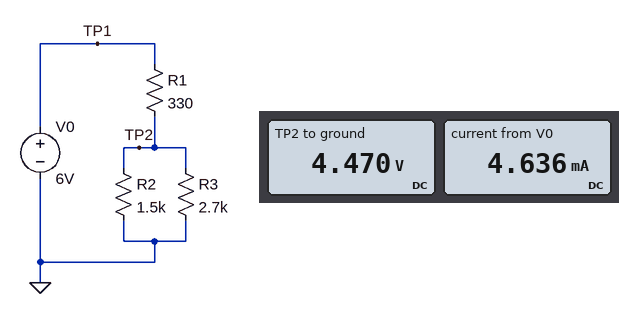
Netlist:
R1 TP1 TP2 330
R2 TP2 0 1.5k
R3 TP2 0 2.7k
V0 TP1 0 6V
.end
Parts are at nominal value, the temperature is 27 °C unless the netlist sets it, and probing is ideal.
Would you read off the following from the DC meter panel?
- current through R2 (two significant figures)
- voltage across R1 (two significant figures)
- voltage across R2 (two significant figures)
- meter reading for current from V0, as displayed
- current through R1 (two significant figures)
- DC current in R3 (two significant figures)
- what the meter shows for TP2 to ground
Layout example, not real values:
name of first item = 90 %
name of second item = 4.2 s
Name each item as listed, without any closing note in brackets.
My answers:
current through R2 = 3.0 mA
voltage across R1 = 1.5 V
voltage across R2 = 4.5 V
meter reading for current from V0, as displayed = 4.636 mA
current through R1 = 4.6 mA
DC current in R3 = 1.7 mA
what the meter shows for TP2 to ground = 4.470 V
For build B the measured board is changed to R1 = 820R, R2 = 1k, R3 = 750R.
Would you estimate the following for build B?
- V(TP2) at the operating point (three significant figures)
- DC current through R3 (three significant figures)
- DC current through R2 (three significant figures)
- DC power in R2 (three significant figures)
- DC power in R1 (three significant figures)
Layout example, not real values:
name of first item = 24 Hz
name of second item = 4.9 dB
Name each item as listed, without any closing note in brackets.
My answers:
V(TP2) at the operating point = 2.06 V
DC current through R3 = 2.75 mA
DC current through R2 = 2.06 mA
DC power in R2 = 4.24 mW
DC power in R1 = 18.9 mW
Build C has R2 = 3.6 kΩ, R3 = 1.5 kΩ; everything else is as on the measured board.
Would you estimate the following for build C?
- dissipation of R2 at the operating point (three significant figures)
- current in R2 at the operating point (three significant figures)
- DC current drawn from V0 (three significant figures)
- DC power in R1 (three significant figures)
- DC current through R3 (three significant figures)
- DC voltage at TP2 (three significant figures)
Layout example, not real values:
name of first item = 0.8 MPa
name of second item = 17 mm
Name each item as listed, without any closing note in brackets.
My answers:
dissipation of R2 at the operating point = 5.81 mW
current in R2 at the operating point = 1.27 mA
DC current drawn from V0 = 4.32 mA
DC power in R1 = 6.16 mW
DC current through R3 = 3.05 mA
DC voltage at TP2 = 4.57 V
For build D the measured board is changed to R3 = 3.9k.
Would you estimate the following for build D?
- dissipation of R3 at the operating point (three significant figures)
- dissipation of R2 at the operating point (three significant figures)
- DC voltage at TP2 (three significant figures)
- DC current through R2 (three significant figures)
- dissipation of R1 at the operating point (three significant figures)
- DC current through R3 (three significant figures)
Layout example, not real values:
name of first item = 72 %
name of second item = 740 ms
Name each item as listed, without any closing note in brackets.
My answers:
dissipation of R3 at the operating point = 5.42 mW
dissipation of R2 at the operating point = 14.1 mW
DC voltage at TP2 = 4.60 V
DC current through R2 = 3.07 mA
dissipation of R1 at the operating point = 5.95 mW
DC current through R3 = 1.18 mA
